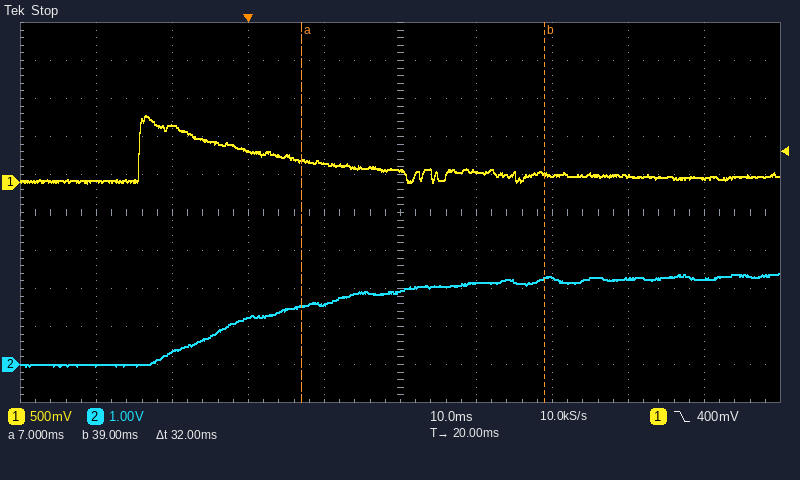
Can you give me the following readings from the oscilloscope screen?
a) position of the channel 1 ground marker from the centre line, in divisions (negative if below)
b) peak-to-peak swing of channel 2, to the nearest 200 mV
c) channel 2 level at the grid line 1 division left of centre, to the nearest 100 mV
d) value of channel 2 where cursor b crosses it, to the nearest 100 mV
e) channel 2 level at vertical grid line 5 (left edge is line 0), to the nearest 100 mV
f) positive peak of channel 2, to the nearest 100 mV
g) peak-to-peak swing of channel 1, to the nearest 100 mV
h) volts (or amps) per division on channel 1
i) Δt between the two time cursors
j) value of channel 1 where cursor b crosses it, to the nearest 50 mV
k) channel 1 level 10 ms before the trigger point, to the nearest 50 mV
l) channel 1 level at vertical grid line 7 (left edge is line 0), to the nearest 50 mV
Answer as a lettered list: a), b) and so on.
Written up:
a) +0.8 div
b) 2.4 V
c) 1.6 V
d) 2.3 V
e) 1.9 V
f) 2.4 V
g) 900 mV
h) 500 mV
i) 32 ms
j) 100 mV
k) 750 mV
l) 100 mV
